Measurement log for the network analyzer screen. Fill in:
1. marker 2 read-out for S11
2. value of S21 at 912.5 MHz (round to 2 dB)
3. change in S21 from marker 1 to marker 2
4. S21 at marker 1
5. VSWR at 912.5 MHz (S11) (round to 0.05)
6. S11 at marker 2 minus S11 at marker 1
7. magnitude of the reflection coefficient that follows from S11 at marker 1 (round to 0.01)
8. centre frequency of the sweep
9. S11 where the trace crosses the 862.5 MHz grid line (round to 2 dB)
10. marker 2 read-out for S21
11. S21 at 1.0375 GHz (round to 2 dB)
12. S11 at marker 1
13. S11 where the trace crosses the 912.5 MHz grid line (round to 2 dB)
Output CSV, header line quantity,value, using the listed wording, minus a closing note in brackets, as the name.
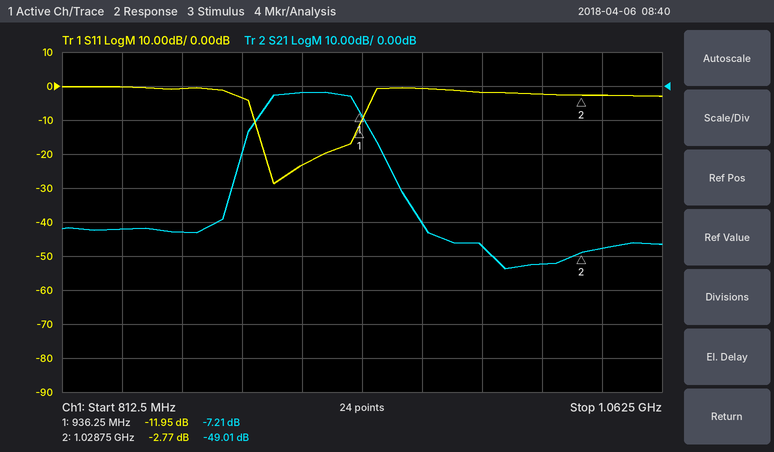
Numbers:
quantity,value
marker 2 read-out for S11,-2.77 dB
value of S21 at 912.5 MHz,-2 dB
change in S21 from marker 1 to marker 2,-41.80 dB
S21 at marker 1,-7.21 dB
VSWR at 912.5 MHz (S11),1.15
S11 at marker 2 minus S11 at marker 1,9.18 dB
magnitude of the reflection coefficient that follows from S11 at marker 1,0.25
centre frequency of the sweep,937.5 MHz
S11 where the trace crosses the 862.5 MHz grid line,0 dB
marker 2 read-out for S21,-49.01 dB
S21 at 1.0375 GHz,-48 dB
S11 at marker 1,-11.95 dB
S11 where the trace crosses the 912.5 MHz grid line,-24 dB
